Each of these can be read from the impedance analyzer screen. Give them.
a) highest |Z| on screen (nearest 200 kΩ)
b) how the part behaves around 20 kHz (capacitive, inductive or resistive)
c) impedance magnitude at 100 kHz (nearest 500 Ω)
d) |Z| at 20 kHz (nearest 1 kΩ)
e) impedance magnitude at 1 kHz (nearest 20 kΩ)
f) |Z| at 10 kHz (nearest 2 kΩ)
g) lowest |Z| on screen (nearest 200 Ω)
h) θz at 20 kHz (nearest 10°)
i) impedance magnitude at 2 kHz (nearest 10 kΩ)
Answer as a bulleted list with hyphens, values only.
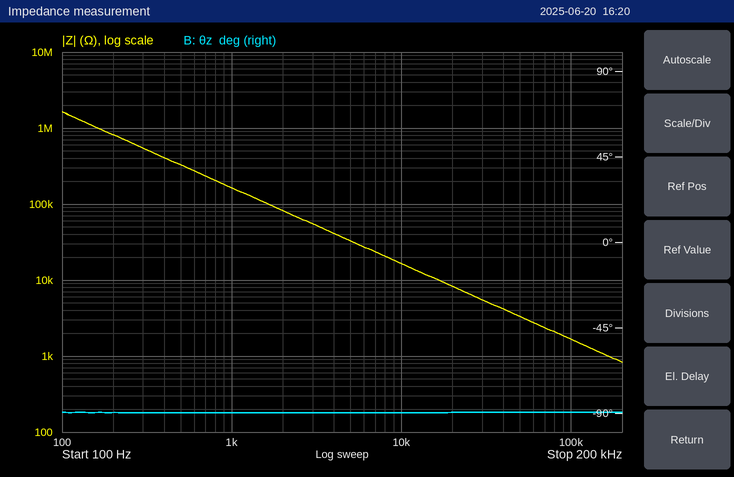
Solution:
- 1.6 MΩ
- capacitive
- 1.5 kΩ
- 8 kΩ
- 160 kΩ
- 16 kΩ
- 800 Ω
- -90°
- 80 kΩ
